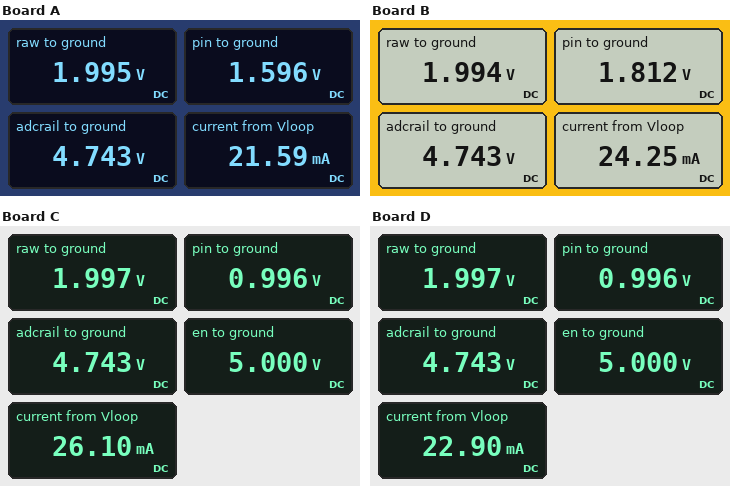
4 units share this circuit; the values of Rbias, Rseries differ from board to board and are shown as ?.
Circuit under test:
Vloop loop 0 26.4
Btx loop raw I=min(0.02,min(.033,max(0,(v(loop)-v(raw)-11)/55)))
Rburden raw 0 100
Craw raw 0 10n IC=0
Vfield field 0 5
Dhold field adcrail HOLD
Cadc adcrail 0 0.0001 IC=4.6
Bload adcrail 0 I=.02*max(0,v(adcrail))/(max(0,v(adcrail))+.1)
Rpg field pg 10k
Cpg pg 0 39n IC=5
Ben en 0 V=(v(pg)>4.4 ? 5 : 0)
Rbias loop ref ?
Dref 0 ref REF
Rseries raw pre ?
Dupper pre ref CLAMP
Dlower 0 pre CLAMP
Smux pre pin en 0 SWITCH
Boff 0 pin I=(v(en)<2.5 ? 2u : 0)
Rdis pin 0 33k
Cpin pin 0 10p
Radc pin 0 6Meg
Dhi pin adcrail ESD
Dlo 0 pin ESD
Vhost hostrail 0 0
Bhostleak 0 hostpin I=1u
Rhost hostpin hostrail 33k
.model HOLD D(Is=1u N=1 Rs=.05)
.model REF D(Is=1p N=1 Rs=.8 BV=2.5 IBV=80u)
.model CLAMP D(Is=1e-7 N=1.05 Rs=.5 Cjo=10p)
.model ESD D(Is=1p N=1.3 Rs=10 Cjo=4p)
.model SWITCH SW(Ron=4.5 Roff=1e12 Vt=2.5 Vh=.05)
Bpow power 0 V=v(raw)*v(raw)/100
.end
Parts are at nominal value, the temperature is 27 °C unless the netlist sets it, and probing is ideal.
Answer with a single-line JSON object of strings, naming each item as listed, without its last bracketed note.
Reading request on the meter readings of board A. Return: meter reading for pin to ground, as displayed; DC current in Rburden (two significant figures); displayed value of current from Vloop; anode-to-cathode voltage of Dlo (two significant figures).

{"meter reading for pin to ground, as displayed": "1.596 V", "DC current in Rburden": "20 mA", "displayed value of current from Vloop": "21.59 mA", "anode-to-cathode voltage of Dlo": "-1.6 V"}
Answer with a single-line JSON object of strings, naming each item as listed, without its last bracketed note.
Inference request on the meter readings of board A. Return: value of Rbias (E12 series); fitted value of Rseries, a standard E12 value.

{"value of Rbias": "15 kΩ", "fitted value of Rseries, a standard E12 value": "8.2 kΩ"}
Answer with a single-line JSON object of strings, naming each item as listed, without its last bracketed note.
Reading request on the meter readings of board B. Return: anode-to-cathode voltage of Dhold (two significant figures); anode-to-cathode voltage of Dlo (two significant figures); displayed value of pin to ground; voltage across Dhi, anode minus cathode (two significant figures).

{"anode-to-cathode voltage of Dhold": "260 mV", "anode-to-cathode voltage of Dlo": "-1.8 V", "displayed value of pin to ground": "1.812 V", "voltage across Dhi, anode minus cathode": "-2.9 V"}
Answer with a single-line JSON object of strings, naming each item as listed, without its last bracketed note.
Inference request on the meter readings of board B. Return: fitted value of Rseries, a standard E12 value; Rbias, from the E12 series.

{"fitted value of Rseries, a standard E12 value": "3.3 kΩ", "Rbias, from the E12 series": "5.6 kΩ"}
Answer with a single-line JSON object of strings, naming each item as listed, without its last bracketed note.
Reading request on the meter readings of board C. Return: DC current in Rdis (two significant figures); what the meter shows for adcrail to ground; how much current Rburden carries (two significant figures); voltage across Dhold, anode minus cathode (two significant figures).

{"DC current in Rdis": "30 µA", "what the meter shows for adcrail to ground": "4.743 V", "how much current Rburden carries": "20 mA", "voltage across Dhold, anode minus cathode": "260 mV"}
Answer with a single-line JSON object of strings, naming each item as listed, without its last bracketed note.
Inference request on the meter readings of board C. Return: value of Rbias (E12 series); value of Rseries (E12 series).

{"value of Rbias": "3.9 kΩ", "value of Rseries": "33 kΩ"}
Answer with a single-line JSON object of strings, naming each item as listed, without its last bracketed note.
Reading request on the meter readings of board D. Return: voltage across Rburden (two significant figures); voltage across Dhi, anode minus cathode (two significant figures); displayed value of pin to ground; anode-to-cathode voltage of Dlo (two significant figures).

{"voltage across Rburden": "2.0 V", "voltage across Dhi, anode minus cathode": "-3.7 V", "displayed value of pin to ground": "0.996 V", "anode-to-cathode voltage of Dlo": "-1.0 V"}
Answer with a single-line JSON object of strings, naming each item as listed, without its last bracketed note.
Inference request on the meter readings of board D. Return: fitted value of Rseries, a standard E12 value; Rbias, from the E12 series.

{"fitted value of Rseries, a standard E12 value": "33 kΩ", "Rbias, from the E12 series": "8.2 kΩ"}
